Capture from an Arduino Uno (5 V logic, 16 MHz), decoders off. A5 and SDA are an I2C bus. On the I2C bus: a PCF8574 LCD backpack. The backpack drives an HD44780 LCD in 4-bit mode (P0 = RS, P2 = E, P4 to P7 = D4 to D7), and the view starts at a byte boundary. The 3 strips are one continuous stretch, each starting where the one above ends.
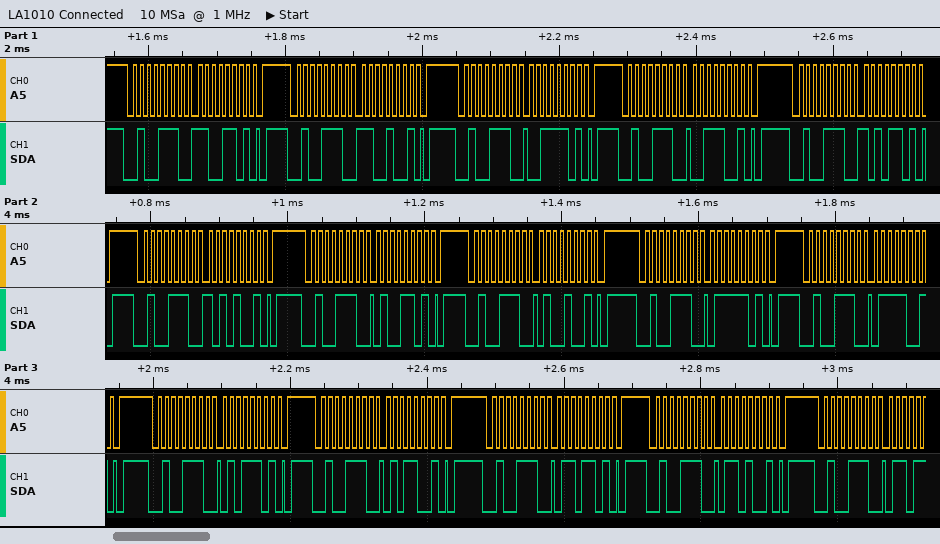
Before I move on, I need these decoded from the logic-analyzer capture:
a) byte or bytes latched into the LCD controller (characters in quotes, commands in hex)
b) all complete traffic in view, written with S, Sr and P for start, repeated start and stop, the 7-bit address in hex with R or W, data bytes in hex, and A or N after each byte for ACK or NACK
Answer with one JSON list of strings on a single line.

["data 0xC3 data 0xA4 'u'", "S 27W A CD A P S 27W A C9 A P S 27W A 3D A P S 27W A 39 A P S 27W A AD A P S 27W A A9 A P S 27W A 4D A P S 27W A 49 A P S 27W A 7D A P S 27W A 79 A P S 27W A 5D A P S 27W A 59 A P S 27W A 6D A P S 27W A 69 A P S 27W A"]
